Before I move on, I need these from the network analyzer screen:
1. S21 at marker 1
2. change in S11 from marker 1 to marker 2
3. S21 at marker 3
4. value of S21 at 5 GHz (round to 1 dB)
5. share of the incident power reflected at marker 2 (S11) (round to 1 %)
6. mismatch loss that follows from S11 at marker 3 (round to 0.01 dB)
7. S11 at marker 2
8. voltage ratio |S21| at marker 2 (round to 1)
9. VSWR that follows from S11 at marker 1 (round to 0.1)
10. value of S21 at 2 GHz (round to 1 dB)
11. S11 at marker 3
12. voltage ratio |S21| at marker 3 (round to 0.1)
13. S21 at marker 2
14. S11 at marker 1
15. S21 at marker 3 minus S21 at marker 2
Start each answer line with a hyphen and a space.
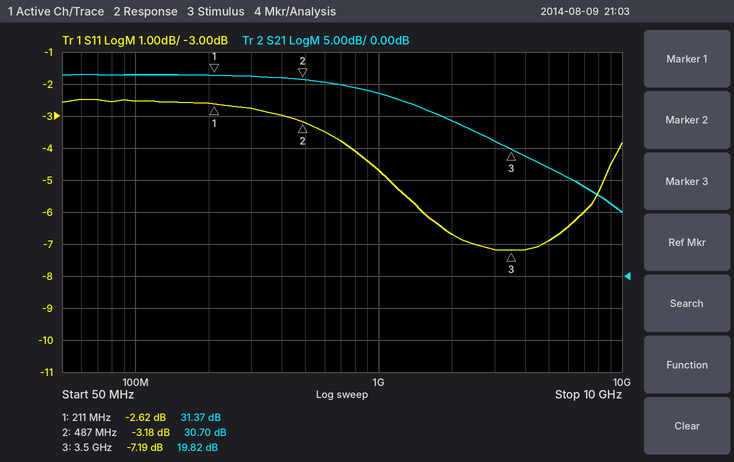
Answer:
- 31.37 dB
- -0.56 dB
- 19.82 dB
- 17 dB
- 48 %
- 0.92 dB
- -3.18 dB
- 34
- 6.7
- 24 dB
- -7.19 dB
- 9.8
- 30.70 dB
- -2.62 dB
- -10.88 dB
